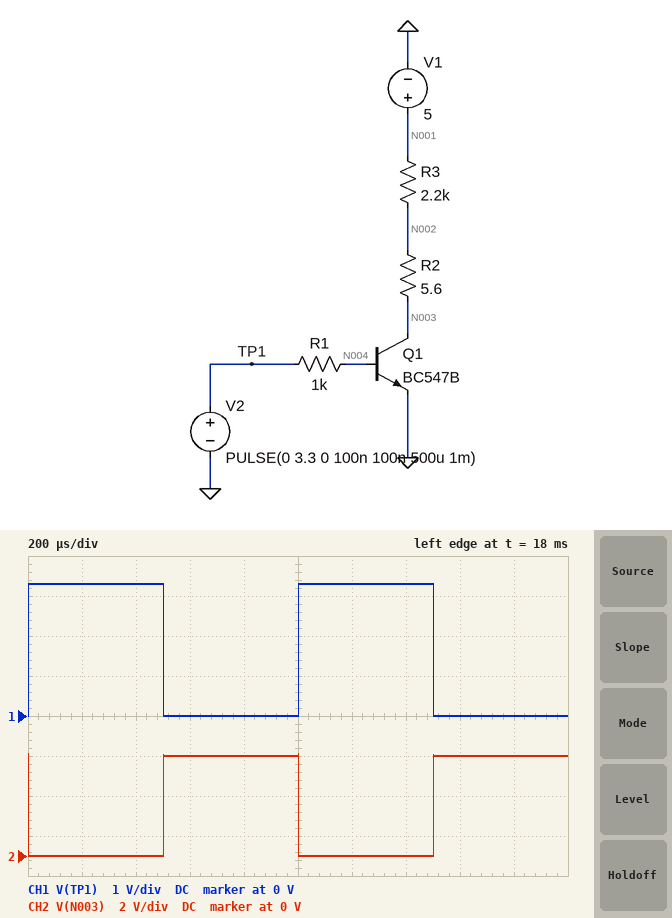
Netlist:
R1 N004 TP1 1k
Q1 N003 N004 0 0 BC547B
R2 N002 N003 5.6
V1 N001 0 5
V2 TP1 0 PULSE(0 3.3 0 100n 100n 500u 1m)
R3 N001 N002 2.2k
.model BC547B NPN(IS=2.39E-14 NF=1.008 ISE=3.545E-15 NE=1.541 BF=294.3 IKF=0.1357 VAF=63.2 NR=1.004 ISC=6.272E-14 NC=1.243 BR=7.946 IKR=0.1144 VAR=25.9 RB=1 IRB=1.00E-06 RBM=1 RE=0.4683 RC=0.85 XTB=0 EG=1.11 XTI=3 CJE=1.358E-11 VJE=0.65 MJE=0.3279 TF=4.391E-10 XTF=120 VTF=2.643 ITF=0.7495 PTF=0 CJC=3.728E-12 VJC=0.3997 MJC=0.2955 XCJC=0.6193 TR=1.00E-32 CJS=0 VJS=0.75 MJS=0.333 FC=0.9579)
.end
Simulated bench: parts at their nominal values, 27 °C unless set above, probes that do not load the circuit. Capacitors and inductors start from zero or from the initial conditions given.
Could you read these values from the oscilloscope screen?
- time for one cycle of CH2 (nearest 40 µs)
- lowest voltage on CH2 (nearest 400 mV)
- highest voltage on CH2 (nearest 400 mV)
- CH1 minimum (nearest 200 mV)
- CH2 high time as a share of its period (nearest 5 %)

1.00 ms
0 V
5.2 V
0 V
50 %
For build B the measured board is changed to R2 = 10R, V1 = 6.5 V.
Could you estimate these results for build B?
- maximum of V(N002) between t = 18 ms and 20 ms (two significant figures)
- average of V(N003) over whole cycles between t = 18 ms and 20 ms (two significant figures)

6.6 V
3.3 V
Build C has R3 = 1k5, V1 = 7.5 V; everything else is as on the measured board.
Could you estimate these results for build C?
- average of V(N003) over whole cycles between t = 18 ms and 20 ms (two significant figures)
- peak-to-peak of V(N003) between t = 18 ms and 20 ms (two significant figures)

3.8 V
7.5 V
